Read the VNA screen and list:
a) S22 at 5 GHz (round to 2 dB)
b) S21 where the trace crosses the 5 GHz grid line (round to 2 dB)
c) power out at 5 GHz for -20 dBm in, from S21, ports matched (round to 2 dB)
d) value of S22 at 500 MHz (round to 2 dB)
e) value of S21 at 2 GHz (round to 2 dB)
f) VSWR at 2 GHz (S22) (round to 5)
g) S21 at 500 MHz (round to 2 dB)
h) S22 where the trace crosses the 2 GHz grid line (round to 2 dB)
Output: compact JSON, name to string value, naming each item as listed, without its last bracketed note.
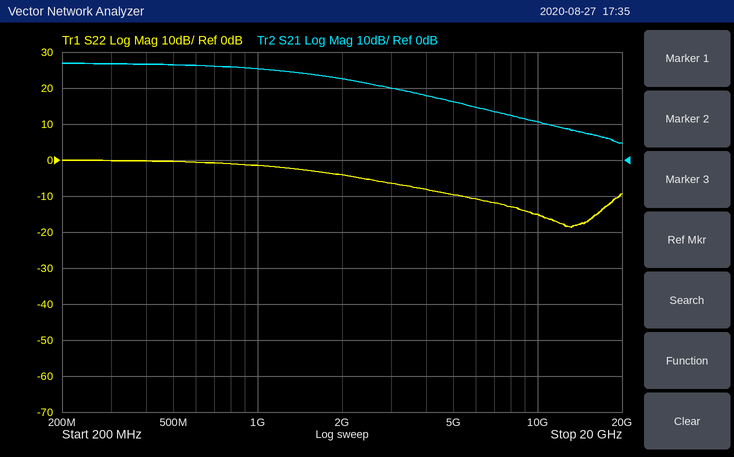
{"S22 at 5 GHz": "-10 dB", "S21 where the trace crosses the 5 GHz grid line": "16 dB", "power out at 5 GHz for -20 dBm in, from S21, ports matched": "-4 dBm", "value of S22 at 500 MHz": "0 dB", "value of S21 at 2 GHz": "22 dB", "VSWR at 2 GHz (S22)": "5", "S21 at 500 MHz": "26 dB", "S22 where the trace crosses the 2 GHz grid line": "-4 dB"}
